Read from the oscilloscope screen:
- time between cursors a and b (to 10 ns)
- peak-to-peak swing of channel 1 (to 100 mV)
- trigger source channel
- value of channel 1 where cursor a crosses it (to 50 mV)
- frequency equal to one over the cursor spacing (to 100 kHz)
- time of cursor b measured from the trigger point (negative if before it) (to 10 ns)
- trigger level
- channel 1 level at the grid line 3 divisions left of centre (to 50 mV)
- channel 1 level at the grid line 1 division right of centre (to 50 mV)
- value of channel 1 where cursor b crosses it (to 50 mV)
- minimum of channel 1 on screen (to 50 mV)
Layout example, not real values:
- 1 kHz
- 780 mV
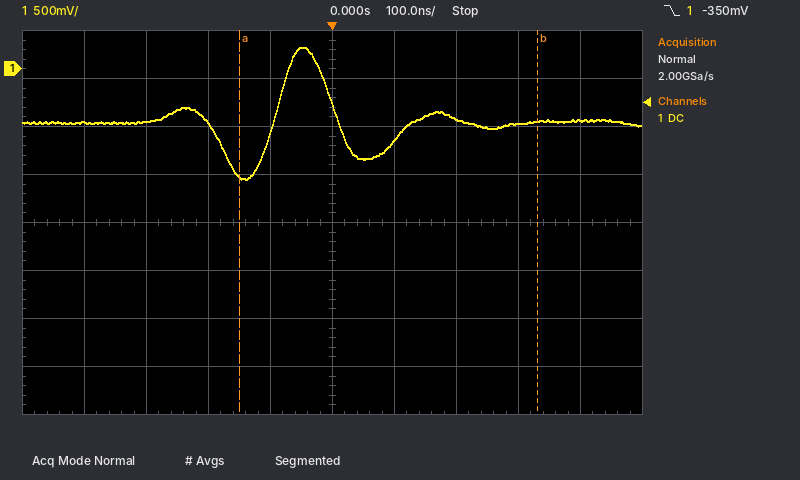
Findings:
- 480 ns
- 1.40 V
- channel 1
- -1.10 V
- 2.1 MHz
- +330 ns
- -350 mV
- -550 mV
- -750 mV
- -550 mV
- -1.15 V
